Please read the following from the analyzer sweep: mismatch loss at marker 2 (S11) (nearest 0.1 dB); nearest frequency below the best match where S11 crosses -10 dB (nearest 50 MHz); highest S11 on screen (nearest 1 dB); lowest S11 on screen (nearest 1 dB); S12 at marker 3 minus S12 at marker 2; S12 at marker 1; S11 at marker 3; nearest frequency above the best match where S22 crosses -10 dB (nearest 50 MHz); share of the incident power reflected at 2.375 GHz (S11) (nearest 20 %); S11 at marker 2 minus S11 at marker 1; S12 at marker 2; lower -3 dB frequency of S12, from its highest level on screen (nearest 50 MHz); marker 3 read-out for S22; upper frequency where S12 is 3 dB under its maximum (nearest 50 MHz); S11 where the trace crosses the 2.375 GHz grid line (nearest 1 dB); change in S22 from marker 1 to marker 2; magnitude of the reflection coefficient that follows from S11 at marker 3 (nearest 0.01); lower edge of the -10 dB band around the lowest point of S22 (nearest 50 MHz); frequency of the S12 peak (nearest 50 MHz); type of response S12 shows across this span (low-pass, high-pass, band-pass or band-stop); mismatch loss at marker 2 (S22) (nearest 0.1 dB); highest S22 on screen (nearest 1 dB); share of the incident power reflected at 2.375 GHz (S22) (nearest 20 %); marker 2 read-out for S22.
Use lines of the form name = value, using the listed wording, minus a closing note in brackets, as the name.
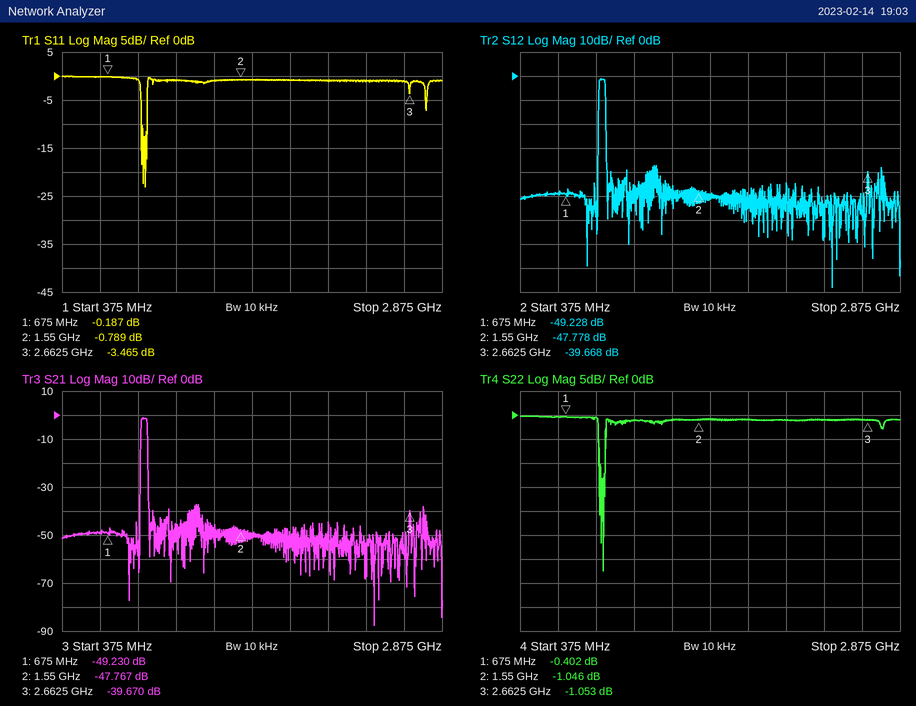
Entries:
mismatch loss at marker 2 (S11) = 7.8 dB
nearest frequency below the best match where S11 crosses -10 dB = 900 MHz
highest S11 on screen = 0 dB
lowest S11 on screen = -23 dB
S12 at marker 3 minus S12 at marker 2 = 8.110 dB
S12 at marker 1 = -49.228 dB
S11 at marker 3 = -3.465 dB
nearest frequency above the best match where S22 crosses -10 dB = 950 MHz
share of the incident power reflected at 2.375 GHz (S11) = 80 %
S11 at marker 2 minus S11 at marker 1 = -0.602 dB
S12 at marker 2 = -47.778 dB
lower -3 dB frequency of S12, from its highest level on screen = 900 MHz
marker 3 read-out for S22 = -1.053 dB
upper frequency where S12 is 3 dB under its maximum = 950 MHz
S11 where the trace crosses the 2.375 GHz grid line = -1 dB
change in S22 from marker 1 to marker 2 = -0.644 dB
magnitude of the reflection coefficient that follows from S11 at marker 3 = 0.67
lower edge of the -10 dB band around the lowest point of S22 = 900 MHz
frequency of the S12 peak = 900 MHz
type of response S12 shows across this span = band-pass
mismatch loss at marker 2 (S22) = 6.7 dB
highest S22 on screen = 0 dB
share of the incident power reflected at 2.375 GHz (S22) = 80 %
marker 2 read-out for S22 = -1.046 dB
